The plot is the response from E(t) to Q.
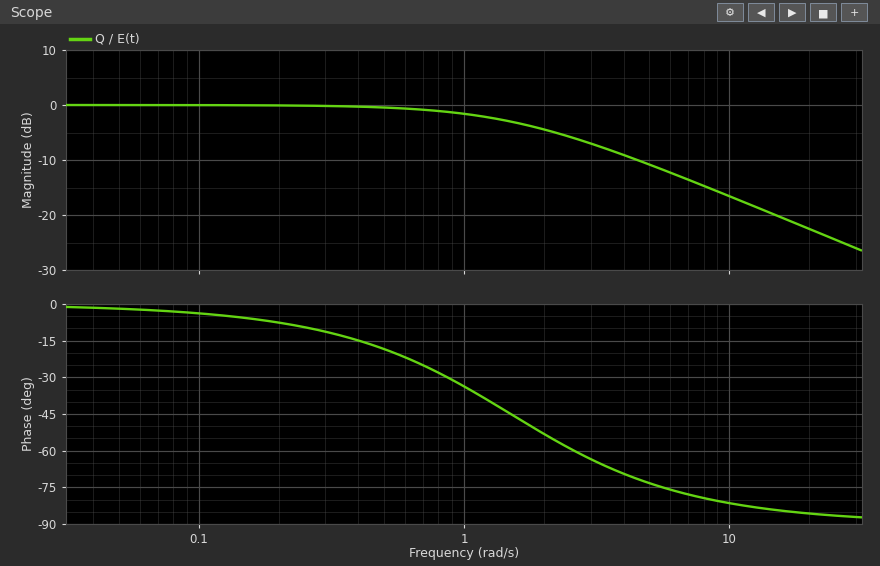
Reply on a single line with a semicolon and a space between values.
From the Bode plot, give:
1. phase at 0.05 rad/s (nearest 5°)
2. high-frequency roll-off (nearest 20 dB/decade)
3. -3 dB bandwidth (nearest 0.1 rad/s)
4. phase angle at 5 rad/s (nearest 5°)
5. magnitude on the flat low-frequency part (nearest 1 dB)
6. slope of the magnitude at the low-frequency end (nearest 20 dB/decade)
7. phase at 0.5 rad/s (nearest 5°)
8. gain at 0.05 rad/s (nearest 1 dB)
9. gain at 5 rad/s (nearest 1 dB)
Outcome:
0°; -20 dB/decade; 1.5 rad/s; -75°; 0 dB; 0 dB/decade; -20°; 0 dB; -11 dB
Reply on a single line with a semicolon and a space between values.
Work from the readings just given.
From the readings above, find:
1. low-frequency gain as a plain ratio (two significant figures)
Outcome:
1.0
